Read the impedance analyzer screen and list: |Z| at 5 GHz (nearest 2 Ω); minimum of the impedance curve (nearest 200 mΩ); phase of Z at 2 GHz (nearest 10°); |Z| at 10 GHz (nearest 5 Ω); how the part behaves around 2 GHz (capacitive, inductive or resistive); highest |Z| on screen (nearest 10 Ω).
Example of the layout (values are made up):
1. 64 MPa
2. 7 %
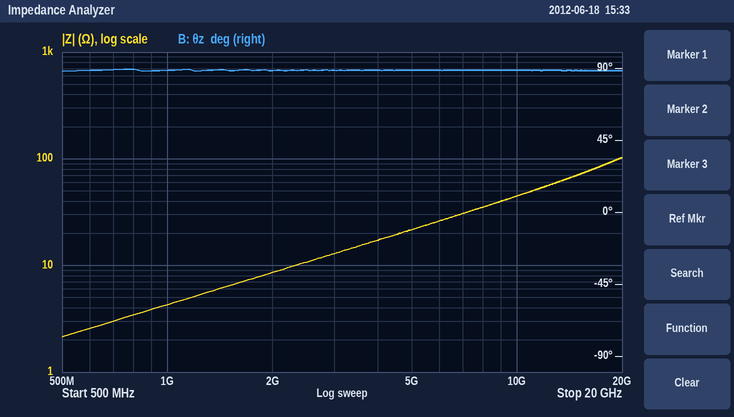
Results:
1. 22 Ω
2. 2.2 Ω
3. 90°
4. 45 Ω
5. inductive
6. 100 Ω
